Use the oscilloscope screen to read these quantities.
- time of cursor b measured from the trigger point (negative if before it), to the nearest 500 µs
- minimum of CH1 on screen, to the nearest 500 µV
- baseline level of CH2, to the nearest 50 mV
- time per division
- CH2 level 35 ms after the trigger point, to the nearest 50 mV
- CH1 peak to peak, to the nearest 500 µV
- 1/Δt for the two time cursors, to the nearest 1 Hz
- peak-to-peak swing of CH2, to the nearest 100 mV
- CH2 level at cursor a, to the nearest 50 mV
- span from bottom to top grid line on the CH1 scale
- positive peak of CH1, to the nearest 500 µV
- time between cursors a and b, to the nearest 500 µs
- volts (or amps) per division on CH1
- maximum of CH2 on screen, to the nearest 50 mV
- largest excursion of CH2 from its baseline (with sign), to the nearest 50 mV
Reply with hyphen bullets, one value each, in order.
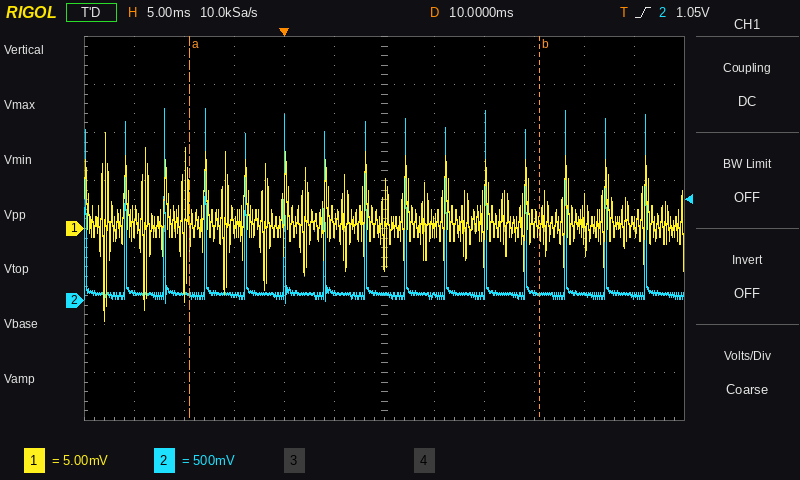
- +25.5 ms
- -9.5 mV
- 50 mV
- 5 ms
- 50 mV
- 19.5 mV
- 29 Hz
- 2.00 V
- 50 mV
- 40 mV
- 10.0 mV
- 35.0 ms
- 5 mV
- 2.00 V
- +1.95 V
